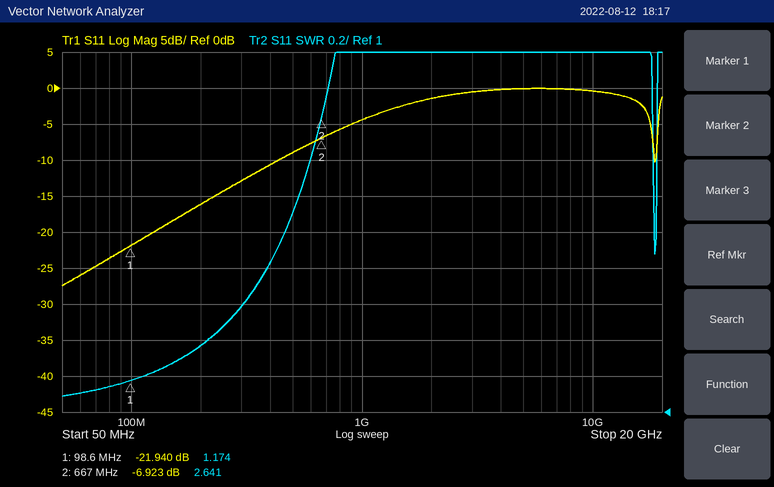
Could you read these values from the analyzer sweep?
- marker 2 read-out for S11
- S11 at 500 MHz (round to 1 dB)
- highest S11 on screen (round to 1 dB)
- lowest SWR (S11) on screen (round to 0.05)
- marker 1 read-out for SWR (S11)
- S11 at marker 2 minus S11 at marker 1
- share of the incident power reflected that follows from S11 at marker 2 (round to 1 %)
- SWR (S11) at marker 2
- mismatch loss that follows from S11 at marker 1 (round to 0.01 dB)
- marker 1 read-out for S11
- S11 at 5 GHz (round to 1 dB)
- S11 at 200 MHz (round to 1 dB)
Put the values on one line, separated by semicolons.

-6.923 dB; -9 dB; 0 dB; 1.10; 1.174; 15.017 dB; 20 %; 2.641; 0.03 dB; -21.940 dB; 0 dB; -16 dB
